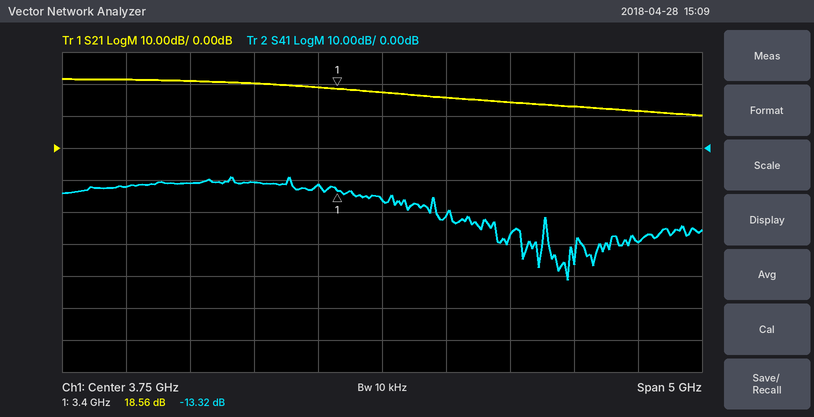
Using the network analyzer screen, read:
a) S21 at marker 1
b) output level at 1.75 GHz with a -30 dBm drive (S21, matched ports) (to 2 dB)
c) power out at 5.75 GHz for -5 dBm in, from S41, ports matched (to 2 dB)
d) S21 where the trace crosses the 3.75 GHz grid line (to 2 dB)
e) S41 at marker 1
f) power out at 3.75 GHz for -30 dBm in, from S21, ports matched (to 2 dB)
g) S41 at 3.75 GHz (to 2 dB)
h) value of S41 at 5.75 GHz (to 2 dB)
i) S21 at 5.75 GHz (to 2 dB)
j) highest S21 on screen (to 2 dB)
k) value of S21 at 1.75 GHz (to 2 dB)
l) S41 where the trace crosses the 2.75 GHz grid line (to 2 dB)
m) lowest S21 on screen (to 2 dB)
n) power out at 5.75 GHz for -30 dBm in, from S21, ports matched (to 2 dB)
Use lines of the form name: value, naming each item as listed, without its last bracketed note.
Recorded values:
S21 at marker 1: 18.56 dB
output level at 1.75 GHz with a -30 dBm drive (S21, matched ports): -8 dBm
power out at 5.75 GHz for -5 dBm in, from S41, ports matched: -34 dBm
S21 where the trace crosses the 3.75 GHz grid line: 18 dB
S41 at marker 1: -13.32 dB
power out at 3.75 GHz for -30 dBm in, from S21, ports matched: -12 dBm
S41 at 3.75 GHz: -16 dB
value of S41 at 5.75 GHz: -30 dB
S21 at 5.75 GHz: 12 dB
highest S21 on screen: 22 dB
value of S21 at 1.75 GHz: 22 dB
S41 where the trace crosses the 2.75 GHz grid line: -10 dB
lowest S21 on screen: 10 dB
power out at 5.75 GHz for -30 dBm in, from S21, ports matched: -18 dBm
